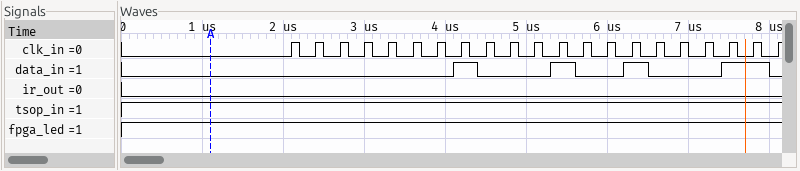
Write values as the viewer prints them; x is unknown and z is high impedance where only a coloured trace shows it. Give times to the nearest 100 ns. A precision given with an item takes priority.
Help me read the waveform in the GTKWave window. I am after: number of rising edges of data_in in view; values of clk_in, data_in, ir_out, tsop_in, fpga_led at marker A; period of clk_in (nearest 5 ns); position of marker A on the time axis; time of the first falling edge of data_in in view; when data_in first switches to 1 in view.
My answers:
4
clk_in=0, data_in=0, ir_out=0, tsop_in=1, fpga_led=1
300 ns
1100 ns
4400 ns
4100 ns
